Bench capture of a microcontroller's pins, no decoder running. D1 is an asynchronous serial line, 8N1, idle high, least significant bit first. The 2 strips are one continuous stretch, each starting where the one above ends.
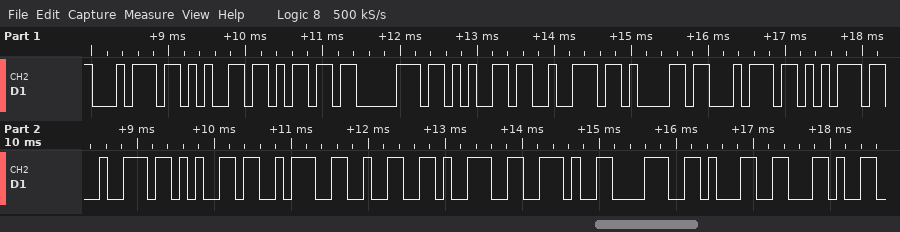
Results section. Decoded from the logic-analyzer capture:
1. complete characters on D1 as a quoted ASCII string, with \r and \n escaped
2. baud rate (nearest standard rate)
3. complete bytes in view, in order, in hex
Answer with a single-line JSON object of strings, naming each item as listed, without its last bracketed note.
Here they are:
{"complete characters on D1 as a quoted ASCII string, with \\r and \\n escaped": "\"temperature:29.81,\"", "baud rate": "9600 baud", "complete bytes in view, in order, in hex": "74 65 6D 70 65 72 61 74 75 72 65 3A 32 39 2E 38 31 2C"}
